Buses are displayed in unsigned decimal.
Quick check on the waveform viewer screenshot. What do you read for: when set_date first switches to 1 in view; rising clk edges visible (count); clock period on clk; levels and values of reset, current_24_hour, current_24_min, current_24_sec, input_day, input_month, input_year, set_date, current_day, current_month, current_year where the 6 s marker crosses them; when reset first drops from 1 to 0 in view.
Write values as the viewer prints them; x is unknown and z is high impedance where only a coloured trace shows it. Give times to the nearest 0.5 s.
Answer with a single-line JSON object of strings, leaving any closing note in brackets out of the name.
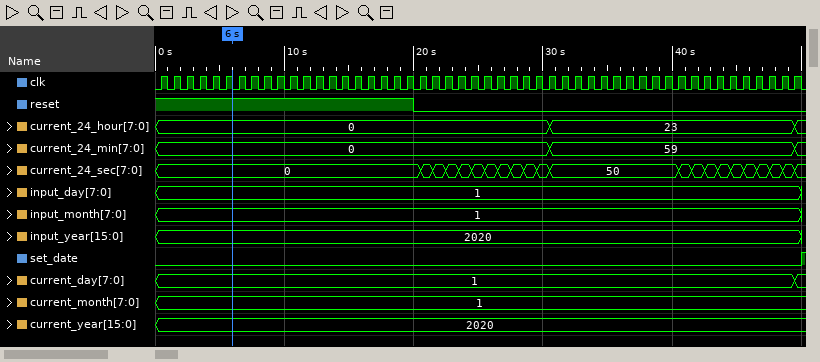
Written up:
{"when set_date first switches to 1 in view": "50 s", "rising clk edges visible": "50", "clock period on clk": "1 s", "levels and values of reset, current_24_hour, current_24_min, current_24_sec, input_day, input_month, input_year, set_date, current_day, current_month, current_year where the 6 s marker crosses them": "reset=1, current_24_hour=0, current_24_min=0, current_24_sec=0, input_day=1, input_month=1, input_year=2020, set_date=0, current_day=1, current_month=1, current_year=2020", "when reset first drops from 1 to 0 in view": "20 s"}
